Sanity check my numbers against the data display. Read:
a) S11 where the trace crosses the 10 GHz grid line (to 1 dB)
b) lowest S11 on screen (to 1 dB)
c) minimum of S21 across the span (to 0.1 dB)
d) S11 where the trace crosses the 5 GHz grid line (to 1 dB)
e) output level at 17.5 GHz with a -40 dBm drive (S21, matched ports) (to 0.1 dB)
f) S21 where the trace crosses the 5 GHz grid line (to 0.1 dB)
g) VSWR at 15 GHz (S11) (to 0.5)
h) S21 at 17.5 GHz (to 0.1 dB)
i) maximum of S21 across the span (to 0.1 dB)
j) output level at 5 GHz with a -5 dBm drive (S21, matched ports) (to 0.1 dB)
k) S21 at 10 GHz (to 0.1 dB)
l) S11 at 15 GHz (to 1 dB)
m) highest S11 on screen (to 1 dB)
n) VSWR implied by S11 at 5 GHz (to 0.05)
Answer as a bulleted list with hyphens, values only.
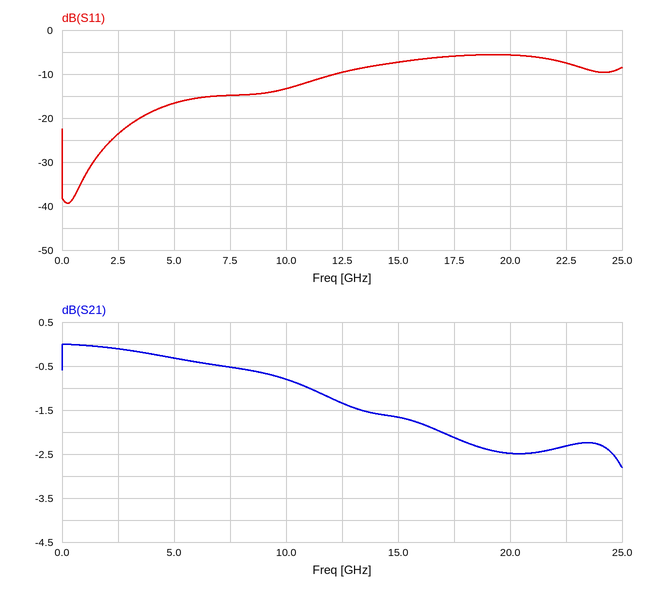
- -13 dB
- -39 dB
- -2.8 dB
- -17 dB
- -42.1 dBm
- -0.3 dB
- 2.5
- -2.1 dB
- 0.0 dB
- -5.3 dBm
- -0.8 dB
- -7 dB
- -6 dB
- 1.35
